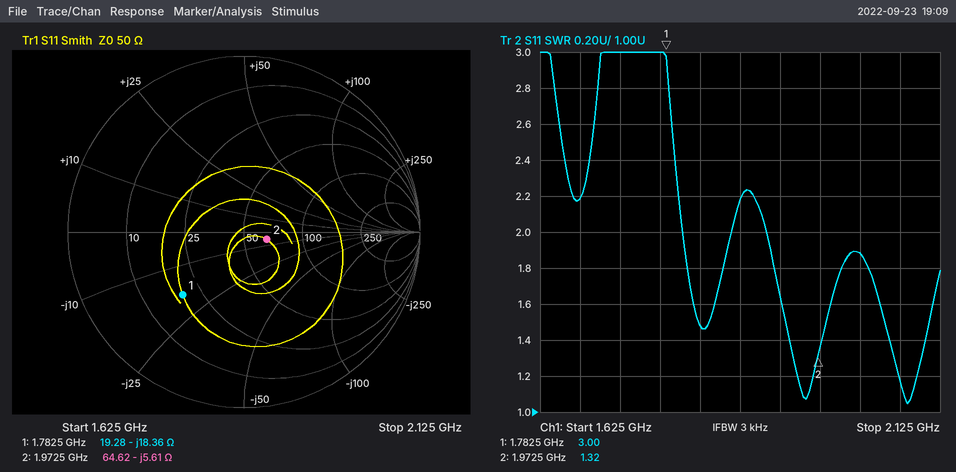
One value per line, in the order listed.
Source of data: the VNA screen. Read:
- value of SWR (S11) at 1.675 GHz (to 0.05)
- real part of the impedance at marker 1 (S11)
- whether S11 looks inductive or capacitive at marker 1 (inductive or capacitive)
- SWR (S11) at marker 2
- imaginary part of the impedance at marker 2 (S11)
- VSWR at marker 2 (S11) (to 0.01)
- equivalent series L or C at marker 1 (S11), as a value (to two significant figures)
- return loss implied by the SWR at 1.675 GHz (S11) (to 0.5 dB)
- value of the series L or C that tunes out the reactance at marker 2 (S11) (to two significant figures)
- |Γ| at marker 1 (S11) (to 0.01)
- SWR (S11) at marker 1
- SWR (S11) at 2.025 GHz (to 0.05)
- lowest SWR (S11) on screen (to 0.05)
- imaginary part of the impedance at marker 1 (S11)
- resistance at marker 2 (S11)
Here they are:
2.20
19.28 Ω
capacitive
1.32
-5.61 Ω
1.32
4.9 pF
8.5 dB
450 pH
0.50
3.00
1.90
1.05
-18.36 Ω
64.62 Ω
